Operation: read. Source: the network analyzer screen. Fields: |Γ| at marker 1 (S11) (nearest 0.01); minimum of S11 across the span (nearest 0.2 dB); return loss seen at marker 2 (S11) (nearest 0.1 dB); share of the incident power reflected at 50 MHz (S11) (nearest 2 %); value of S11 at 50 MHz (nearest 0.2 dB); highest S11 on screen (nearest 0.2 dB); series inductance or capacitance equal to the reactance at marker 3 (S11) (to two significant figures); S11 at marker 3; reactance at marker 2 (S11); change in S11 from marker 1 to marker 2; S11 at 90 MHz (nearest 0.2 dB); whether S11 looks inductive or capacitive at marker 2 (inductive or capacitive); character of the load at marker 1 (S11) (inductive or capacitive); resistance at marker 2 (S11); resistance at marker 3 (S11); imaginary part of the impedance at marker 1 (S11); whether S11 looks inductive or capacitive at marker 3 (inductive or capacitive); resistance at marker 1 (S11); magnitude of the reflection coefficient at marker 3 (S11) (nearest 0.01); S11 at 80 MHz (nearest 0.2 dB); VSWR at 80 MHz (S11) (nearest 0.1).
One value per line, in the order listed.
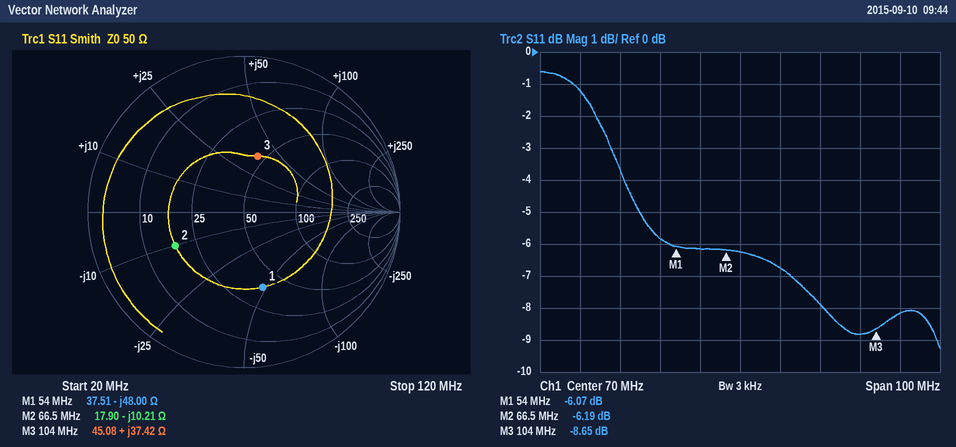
0.50
-9.2 dB
6.2 dB
26 %
-5.8 dB
-0.6 dB
57 nH
-8.65 dB
-10.21 Ω
-0.12 dB
-7.8 dB
capacitive
capacitive
17.90 Ω
45.08 Ω
-48.00 Ω
inductive
37.51 Ω
0.37
-6.8 dB
2.7
